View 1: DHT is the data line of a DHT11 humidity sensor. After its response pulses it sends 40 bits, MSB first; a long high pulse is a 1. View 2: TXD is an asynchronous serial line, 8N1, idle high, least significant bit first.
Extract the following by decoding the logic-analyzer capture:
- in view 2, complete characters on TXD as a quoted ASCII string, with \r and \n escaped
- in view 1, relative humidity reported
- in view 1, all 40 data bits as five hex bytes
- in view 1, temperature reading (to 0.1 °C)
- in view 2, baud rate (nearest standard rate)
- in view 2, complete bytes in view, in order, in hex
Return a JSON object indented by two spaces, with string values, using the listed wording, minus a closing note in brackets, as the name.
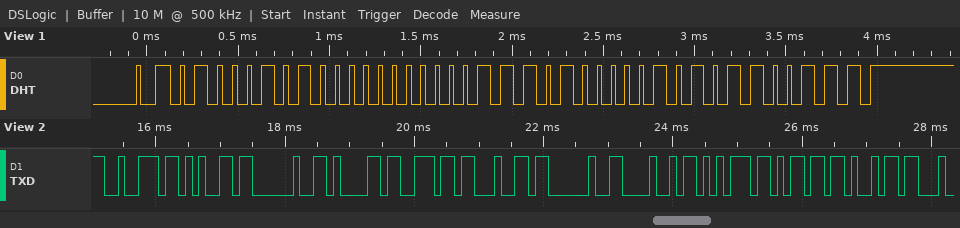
{
  "in view 2, complete characters on TXD as a quoted ASCII string, with \\r and \\n escaped": "\"re and Humi\"",
  "in view 1, relative humidity reported": "69 %",
  "in view 1, all 40 data bits as five hex bytes": "45 00 1D 05 67",
  "in view 1, temperature reading": "29.5 °C",
  "in view 2, baud rate": "9600 baud",
  "in view 2, complete bytes in view, in order, in hex": "0x72 0x65 0x20 0x61 0x6E 0x64 0x20 0x48 0x75 0x6D 0x69"
}
